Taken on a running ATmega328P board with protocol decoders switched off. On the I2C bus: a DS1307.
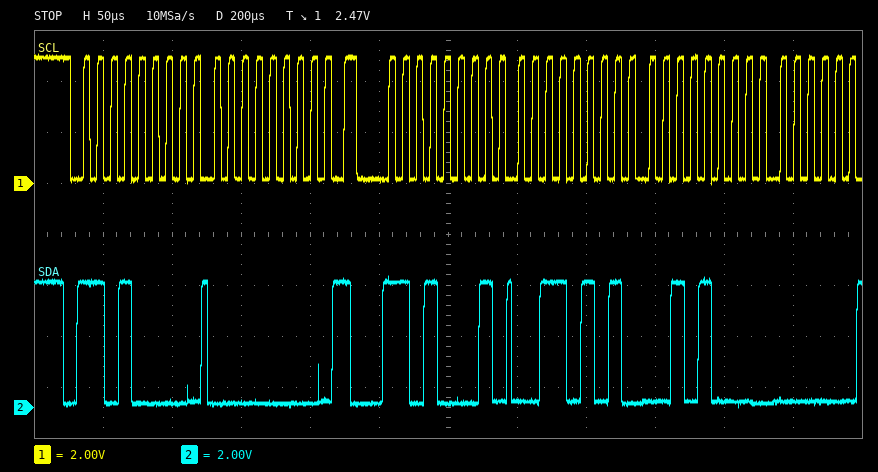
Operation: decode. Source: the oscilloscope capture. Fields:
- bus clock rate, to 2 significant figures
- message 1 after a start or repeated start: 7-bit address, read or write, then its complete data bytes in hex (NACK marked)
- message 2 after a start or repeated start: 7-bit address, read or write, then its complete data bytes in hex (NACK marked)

100 kHz
0x68 write: 00
0x68 read: 35 28
